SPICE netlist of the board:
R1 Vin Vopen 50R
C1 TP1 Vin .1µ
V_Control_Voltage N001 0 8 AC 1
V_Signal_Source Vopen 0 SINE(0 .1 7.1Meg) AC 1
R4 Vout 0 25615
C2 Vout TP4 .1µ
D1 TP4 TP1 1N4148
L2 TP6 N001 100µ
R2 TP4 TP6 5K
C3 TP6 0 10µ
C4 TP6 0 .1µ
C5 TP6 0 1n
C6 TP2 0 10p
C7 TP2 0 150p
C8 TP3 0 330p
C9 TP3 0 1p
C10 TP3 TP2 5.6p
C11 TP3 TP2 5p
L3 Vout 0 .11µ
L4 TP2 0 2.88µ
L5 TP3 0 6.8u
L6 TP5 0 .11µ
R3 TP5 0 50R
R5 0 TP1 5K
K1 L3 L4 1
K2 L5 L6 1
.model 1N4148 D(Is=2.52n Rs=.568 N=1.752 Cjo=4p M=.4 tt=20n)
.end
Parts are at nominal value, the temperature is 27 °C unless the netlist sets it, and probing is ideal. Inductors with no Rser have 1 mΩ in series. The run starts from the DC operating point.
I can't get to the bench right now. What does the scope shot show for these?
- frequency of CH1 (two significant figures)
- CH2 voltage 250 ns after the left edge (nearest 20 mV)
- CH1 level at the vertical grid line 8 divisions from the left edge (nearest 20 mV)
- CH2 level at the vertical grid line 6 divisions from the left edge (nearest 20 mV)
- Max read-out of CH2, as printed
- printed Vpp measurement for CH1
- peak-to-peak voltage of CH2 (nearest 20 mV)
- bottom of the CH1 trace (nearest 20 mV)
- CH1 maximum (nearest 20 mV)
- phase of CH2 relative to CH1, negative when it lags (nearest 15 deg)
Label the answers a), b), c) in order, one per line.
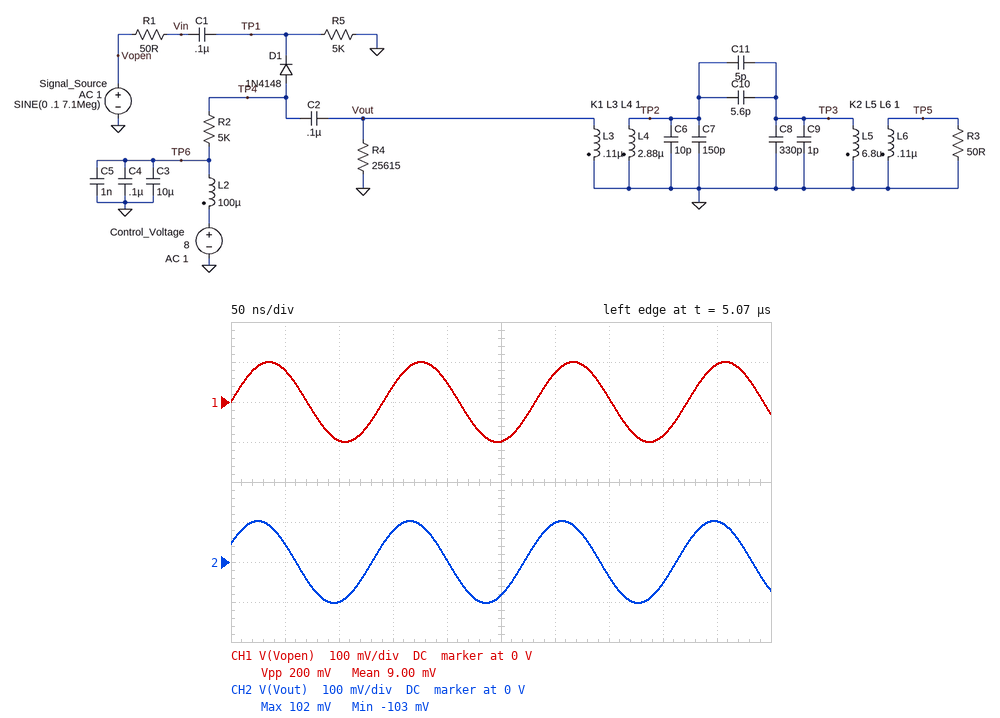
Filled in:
a) 7.1 MHz
b) -80 mV
c) -80 mV
d) 100 mV
e) 102 mV
f) 200 mV
g) 200 mV
h) -100 mV
i) 100 mV
j) 30 deg
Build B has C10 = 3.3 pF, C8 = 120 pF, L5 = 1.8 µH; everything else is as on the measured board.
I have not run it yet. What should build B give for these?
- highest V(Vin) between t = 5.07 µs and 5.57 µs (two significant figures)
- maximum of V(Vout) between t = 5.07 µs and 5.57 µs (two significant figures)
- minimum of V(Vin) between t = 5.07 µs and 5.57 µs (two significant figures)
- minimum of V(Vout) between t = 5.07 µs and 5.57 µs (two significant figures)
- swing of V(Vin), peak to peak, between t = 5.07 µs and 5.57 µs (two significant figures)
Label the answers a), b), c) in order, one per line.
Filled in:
a) 81 mV
b) 99 mV
c) -85 mV
d) -99 mV
e) 170 mV
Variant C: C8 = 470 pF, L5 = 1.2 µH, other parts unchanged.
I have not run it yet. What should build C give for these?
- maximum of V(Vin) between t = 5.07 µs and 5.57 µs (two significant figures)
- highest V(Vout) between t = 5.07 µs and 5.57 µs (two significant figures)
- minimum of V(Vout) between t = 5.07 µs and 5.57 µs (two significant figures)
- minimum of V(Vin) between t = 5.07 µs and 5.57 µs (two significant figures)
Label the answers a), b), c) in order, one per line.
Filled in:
a) 81 mV
b) 93 mV
c) -93 mV
d) -85 mV
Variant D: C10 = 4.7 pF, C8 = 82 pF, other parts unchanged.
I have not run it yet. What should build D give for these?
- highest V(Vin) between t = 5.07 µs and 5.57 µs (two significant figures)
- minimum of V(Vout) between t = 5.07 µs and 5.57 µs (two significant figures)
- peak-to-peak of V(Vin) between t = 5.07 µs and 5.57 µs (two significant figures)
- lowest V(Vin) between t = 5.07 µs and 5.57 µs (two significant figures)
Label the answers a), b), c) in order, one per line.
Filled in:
a) 62 mV
b) -76 mV
c) 130 mV
d) -69 mV
